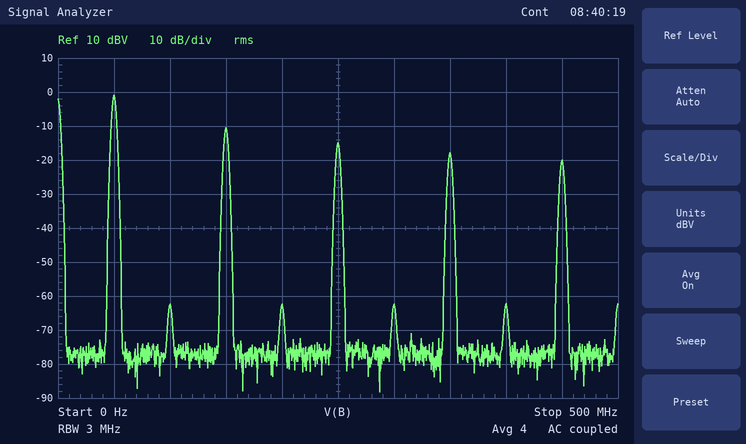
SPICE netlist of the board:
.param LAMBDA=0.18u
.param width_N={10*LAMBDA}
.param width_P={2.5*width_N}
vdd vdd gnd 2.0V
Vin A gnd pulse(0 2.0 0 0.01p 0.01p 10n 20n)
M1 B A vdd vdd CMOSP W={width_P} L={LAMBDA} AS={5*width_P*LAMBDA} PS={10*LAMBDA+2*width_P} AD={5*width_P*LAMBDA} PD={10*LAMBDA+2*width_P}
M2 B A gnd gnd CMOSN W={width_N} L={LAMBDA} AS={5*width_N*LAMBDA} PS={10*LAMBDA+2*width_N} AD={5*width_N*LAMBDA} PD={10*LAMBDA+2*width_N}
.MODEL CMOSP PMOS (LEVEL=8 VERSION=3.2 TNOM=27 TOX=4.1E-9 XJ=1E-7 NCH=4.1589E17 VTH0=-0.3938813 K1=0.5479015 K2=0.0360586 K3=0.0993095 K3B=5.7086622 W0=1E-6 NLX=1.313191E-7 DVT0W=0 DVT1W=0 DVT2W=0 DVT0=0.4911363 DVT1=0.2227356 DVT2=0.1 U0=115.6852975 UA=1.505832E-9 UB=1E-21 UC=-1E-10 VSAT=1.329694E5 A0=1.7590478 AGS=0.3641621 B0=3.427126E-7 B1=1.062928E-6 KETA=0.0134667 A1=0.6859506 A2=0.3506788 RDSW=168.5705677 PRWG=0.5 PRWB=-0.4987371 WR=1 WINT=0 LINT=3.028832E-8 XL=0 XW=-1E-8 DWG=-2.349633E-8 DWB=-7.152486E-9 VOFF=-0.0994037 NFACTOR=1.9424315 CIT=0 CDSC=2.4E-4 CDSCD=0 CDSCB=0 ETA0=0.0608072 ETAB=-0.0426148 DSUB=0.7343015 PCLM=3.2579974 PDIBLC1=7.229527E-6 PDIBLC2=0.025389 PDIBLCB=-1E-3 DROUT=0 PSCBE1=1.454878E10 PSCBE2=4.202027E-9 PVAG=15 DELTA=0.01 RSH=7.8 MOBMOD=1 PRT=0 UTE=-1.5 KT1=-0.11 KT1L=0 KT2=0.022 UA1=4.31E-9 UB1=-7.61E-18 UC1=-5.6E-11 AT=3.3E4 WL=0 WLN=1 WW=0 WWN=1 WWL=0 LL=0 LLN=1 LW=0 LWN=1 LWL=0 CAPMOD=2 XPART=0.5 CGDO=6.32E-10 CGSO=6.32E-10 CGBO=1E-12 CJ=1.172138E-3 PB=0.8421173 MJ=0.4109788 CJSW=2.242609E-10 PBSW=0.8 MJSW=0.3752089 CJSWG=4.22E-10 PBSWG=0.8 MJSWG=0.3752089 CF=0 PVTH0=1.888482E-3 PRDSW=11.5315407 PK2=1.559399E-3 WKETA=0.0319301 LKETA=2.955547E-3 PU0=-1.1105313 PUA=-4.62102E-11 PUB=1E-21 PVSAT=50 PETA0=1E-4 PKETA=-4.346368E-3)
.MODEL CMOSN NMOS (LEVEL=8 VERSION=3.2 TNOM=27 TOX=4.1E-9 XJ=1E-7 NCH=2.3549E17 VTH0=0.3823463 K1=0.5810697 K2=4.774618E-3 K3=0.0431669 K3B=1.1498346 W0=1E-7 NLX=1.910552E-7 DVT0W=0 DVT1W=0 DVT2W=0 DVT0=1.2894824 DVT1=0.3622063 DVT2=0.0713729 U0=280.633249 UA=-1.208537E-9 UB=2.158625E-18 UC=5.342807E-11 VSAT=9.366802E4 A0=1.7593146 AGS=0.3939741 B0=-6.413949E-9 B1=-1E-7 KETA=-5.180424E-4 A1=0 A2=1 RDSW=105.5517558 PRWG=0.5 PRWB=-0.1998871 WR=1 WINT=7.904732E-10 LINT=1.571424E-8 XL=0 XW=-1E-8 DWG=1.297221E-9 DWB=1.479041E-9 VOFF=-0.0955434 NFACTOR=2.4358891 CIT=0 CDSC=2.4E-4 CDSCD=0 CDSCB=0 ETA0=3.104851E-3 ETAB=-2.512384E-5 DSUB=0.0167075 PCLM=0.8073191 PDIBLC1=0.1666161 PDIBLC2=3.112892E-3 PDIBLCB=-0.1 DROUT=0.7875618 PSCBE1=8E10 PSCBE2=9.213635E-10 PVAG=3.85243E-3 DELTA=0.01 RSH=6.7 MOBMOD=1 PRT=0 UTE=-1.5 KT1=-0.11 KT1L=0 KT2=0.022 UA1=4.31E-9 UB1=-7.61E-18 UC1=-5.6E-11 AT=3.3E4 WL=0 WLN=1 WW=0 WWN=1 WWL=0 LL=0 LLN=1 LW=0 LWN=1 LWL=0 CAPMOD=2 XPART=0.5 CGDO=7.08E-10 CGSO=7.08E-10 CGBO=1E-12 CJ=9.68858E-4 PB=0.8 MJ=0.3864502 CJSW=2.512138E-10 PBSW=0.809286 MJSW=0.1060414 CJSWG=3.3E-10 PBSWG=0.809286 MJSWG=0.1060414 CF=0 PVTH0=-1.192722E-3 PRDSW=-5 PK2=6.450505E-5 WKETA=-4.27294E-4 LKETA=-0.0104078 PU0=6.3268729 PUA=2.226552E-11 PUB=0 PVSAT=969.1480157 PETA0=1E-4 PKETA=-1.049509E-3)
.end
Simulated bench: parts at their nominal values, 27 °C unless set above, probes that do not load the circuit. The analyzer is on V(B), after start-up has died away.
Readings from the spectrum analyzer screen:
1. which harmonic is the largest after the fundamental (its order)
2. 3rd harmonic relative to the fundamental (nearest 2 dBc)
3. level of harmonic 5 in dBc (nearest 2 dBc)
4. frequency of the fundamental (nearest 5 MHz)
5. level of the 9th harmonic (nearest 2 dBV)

3
-10 dBc
-14 dBc
50 MHz
-20 dBV
